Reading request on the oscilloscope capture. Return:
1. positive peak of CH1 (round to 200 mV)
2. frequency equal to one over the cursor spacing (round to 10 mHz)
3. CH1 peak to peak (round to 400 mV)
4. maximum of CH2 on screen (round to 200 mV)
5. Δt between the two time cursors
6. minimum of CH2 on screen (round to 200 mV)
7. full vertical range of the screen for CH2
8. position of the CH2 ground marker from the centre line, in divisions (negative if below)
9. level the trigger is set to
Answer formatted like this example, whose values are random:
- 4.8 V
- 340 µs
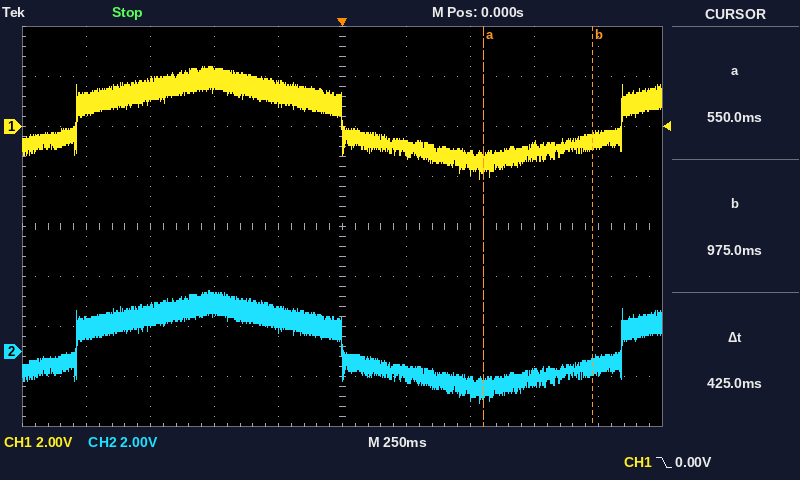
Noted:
- 2.4 V
- 2.35 Hz
- 4.4 V
- 2.4 V
- 425 ms
- -2.0 V
- 16 V
- -2.5 div
- 0.00 V
